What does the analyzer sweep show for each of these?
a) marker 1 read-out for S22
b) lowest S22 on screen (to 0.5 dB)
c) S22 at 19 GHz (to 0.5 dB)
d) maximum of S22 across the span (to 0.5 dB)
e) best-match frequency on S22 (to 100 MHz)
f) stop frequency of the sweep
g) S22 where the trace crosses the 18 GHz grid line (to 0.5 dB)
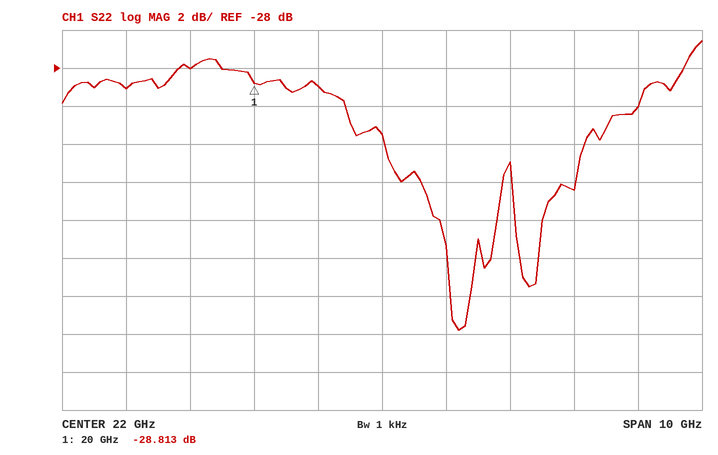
-28.813 dB
-42.0 dB
-28.0 dB
-26.5 dB
23.2 GHz
27 GHz
-29.0 dB
